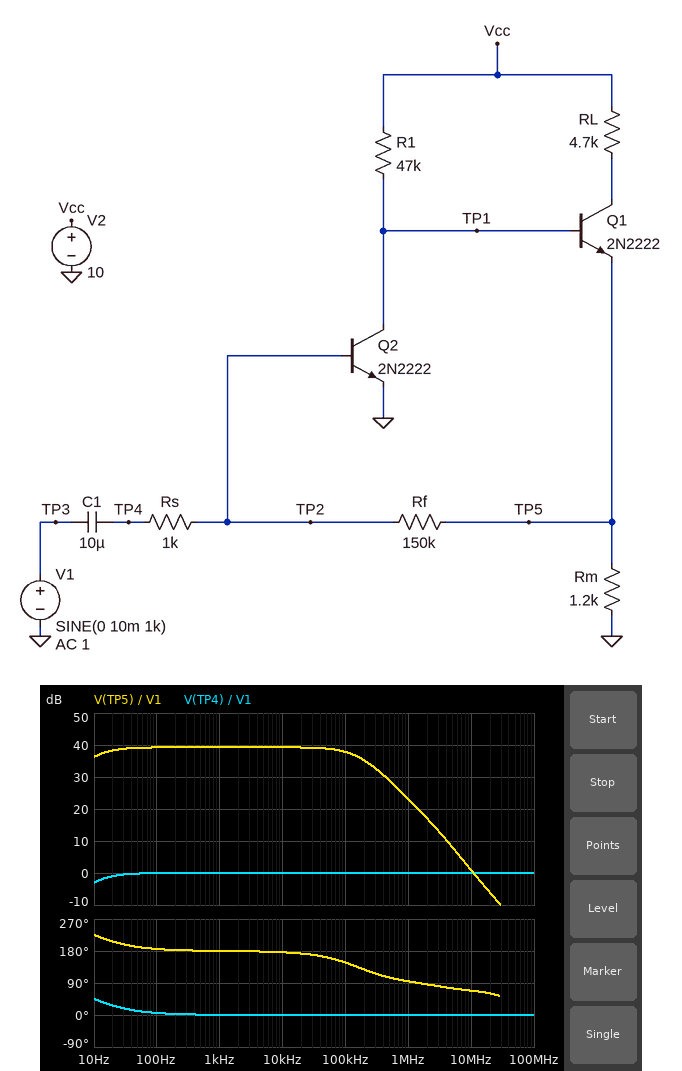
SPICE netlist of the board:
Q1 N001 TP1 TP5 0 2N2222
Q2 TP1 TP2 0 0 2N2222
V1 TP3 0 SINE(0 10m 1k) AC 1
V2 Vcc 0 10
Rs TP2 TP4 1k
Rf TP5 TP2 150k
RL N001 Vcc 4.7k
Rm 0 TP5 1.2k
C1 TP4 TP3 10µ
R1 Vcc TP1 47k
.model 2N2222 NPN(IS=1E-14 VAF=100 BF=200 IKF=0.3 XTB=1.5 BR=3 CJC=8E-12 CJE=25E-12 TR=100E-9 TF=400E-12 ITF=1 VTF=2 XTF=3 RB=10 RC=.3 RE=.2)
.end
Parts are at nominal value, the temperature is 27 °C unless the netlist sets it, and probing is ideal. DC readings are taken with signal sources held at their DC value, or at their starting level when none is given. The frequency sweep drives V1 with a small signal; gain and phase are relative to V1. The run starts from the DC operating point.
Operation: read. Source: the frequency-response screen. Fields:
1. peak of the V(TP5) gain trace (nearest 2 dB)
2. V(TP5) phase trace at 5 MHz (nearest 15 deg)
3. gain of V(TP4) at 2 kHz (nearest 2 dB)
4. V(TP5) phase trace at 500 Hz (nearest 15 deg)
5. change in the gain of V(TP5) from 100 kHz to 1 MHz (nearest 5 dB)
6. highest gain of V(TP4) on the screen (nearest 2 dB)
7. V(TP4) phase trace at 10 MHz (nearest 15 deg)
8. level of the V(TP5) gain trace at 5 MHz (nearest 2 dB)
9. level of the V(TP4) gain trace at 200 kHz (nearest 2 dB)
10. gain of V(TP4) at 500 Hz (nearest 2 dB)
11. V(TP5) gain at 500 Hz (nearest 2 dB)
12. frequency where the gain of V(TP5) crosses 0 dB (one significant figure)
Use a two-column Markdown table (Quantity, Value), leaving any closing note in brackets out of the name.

| Quantity | Value |
|---|---|
| peak of the V(TP5) gain trace | 40 dB |
| V(TP5) phase trace at 5 MHz | 75 deg |
| gain of V(TP4) at 2 kHz | 0 dB |
| V(TP5) phase trace at 500 Hz | 180 deg |
| change in the gain of V(TP5) from 100 kHz to 1 MHz | -15 dB |
| highest gain of V(TP4) on the screen | 0 dB |
| V(TP4) phase trace at 10 MHz | 0 deg |
| level of the V(TP5) gain trace at 5 MHz | 8 dB |
| level of the V(TP4) gain trace at 200 kHz | 0 dB |
| gain of V(TP4) at 500 Hz | 0 dB |
| V(TP5) gain at 500 Hz | 40 dB |
| frequency where the gain of V(TP5) crosses 0 dB | 10 MHz |
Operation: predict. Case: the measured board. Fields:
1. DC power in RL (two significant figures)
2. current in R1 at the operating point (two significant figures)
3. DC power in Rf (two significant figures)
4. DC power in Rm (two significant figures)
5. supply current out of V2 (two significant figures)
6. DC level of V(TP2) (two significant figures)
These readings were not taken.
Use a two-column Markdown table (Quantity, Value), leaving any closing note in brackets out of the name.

| Quantity | Value |
|---|---|
| DC power in RL | 1.8 mW |
| current in R1 at the operating point | 180 µA |
| DC power in Rf | 120 nW |
| DC power in Rm | 460 µW |
| supply current out of V2 | 800 µA |
| DC level of V(TP2) | 610 mV |
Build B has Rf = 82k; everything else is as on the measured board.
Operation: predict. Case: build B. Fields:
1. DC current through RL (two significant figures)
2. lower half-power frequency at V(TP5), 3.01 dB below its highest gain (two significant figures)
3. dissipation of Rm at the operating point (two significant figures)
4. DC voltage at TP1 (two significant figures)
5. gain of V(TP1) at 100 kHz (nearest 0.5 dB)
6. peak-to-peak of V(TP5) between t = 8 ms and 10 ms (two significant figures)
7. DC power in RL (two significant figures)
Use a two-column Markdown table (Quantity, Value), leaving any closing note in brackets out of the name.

| Quantity | Value |
|---|---|
| DC current through RL | 570 µA |
| lower half-power frequency at V(TP5), 3.01 dB below its highest gain | 12 Hz |
| dissipation of Rm at the operating point | 390 µW |
| DC voltage at TP1 | 1.3 V |
| gain of V(TP1) at 100 kHz | 35.5 dB |
| peak-to-peak of V(TP5) between t = 8 ms and 10 ms | 1.2 V |
| DC power in RL | 1.5 mW |
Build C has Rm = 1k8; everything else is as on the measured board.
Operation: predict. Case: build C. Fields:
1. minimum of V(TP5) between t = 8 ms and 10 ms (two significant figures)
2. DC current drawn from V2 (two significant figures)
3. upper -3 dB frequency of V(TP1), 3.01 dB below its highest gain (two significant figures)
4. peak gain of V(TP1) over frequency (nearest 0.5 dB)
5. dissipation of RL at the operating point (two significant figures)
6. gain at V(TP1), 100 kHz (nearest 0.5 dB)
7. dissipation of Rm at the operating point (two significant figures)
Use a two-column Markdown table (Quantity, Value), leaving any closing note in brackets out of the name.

| Quantity | Value |
|---|---|
| minimum of V(TP5) between t = 8 ms and 10 ms | 6.7 mV |
| DC current drawn from V2 | 600 µA |
| upper -3 dB frequency of V(TP1), 3.01 dB below its highest gain | 170 kHz |
| peak gain of V(TP1) over frequency | 40.0 dB |
| dissipation of RL at the operating point | 800 µW |
| gain at V(TP1), 100 kHz | 38.5 dB |
| dissipation of Rm at the operating point | 310 µW |
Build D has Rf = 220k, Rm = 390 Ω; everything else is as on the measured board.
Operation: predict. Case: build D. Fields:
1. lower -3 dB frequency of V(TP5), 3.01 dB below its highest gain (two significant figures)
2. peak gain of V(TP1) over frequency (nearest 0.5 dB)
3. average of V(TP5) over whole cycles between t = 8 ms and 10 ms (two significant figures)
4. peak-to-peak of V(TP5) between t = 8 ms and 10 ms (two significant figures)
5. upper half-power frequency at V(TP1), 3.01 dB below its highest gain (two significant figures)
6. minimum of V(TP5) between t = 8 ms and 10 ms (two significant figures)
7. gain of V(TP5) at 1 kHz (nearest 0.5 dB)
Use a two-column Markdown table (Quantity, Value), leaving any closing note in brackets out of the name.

| Quantity | Value |
|---|---|
| lower -3 dB frequency of V(TP5), 3.01 dB below its highest gain | 690 mHz |
| peak gain of V(TP1) over frequency | 9.0 dB |
| average of V(TP5) over whole cycles between t = 8 ms and 10 ms | 640 mV |
| peak-to-peak of V(TP5) between t = 8 ms and 10 ms | 600 mV |
| upper half-power frequency at V(TP1), 3.01 dB below its highest gain | 1.3 MHz |
| minimum of V(TP5) between t = 8 ms and 10 ms | 190 mV |
| gain of V(TP5) at 1 kHz | 8.0 dB |
